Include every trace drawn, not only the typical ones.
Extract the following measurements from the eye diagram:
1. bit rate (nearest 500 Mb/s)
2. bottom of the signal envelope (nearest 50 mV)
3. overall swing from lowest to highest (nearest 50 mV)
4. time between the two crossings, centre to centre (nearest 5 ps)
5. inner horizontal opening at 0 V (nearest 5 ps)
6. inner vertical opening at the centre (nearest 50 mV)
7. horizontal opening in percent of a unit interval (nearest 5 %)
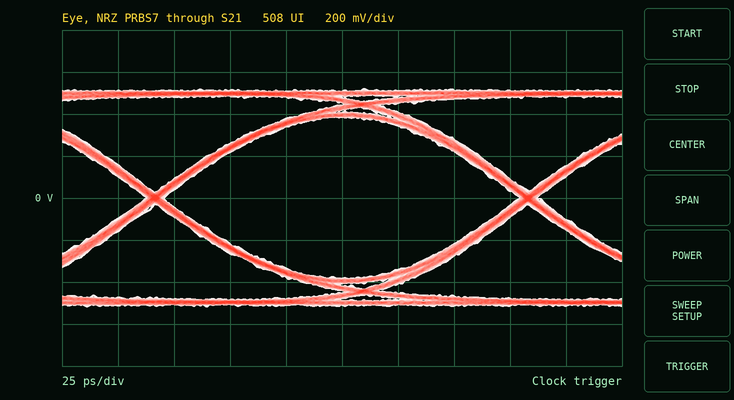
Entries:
6.0 Gb/s
-500 mV
1.05 V
165 ps
160 ps
750 mV
95 %
